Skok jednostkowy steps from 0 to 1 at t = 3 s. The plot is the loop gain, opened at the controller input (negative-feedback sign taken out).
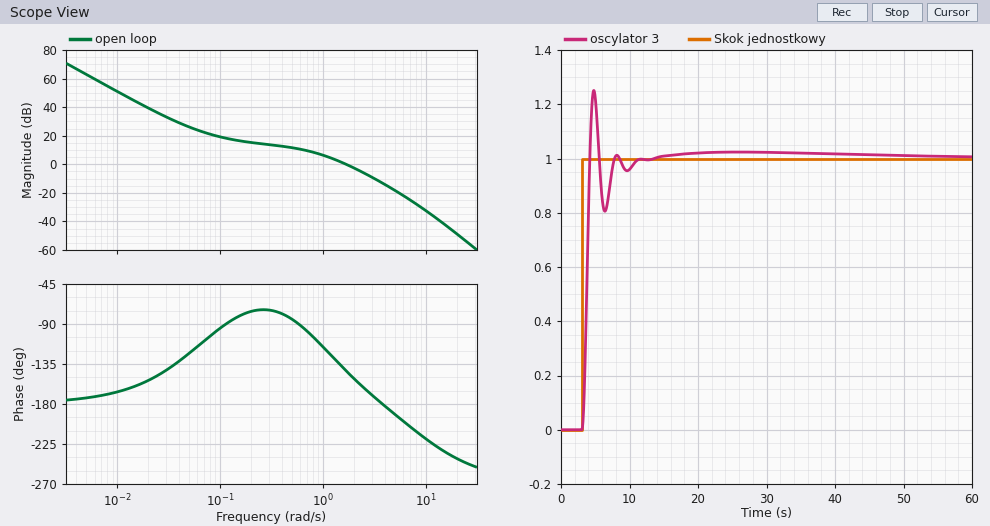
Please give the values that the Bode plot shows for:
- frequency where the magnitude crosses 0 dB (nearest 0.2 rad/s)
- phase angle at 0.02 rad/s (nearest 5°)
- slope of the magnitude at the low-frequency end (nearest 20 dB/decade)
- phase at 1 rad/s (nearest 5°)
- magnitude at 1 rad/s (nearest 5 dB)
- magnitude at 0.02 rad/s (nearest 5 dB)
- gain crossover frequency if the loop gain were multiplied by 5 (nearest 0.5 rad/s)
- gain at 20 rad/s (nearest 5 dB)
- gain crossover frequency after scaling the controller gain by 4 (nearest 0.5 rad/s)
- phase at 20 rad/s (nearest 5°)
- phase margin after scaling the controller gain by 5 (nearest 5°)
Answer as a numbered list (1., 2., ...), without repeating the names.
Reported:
1. 1.6 rad/s
2. -155°
3. -40 dB/decade
4. -115°
5. 5 dB
6. 40 dB
7. 4.0 rad/s
8. -50 dB
9. 3.5 rad/s
10. -240°
11. 0°
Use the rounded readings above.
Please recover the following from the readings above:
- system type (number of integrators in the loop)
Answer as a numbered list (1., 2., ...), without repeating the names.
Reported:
1. 2
